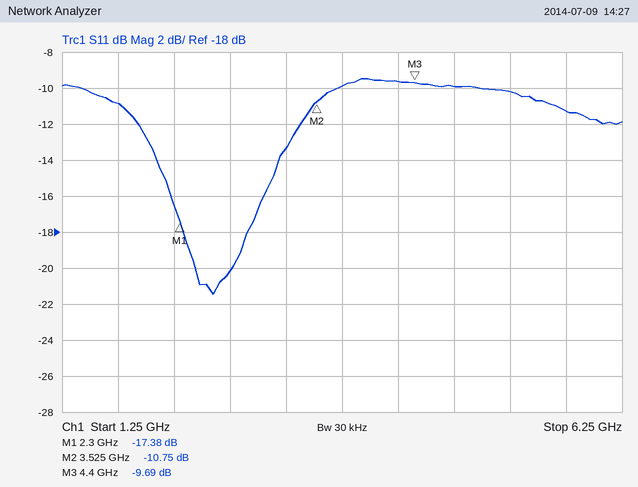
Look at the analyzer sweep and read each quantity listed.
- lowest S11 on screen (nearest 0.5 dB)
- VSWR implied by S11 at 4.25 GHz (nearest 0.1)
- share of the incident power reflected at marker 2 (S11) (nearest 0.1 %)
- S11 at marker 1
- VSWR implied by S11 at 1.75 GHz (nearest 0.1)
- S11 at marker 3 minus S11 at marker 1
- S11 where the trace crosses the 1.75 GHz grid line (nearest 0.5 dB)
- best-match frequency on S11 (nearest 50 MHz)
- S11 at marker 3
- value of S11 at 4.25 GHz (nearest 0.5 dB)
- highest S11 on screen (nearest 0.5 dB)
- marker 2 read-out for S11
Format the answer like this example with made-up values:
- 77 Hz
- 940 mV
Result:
- -21.5 dB
- 2.0
- 8.4 %
- -17.38 dB
- 1.8
- 7.69 dB
- -11.0 dB
- 2.60 GHz
- -9.69 dB
- -9.5 dB
- -9.5 dB
- -10.75 dB
